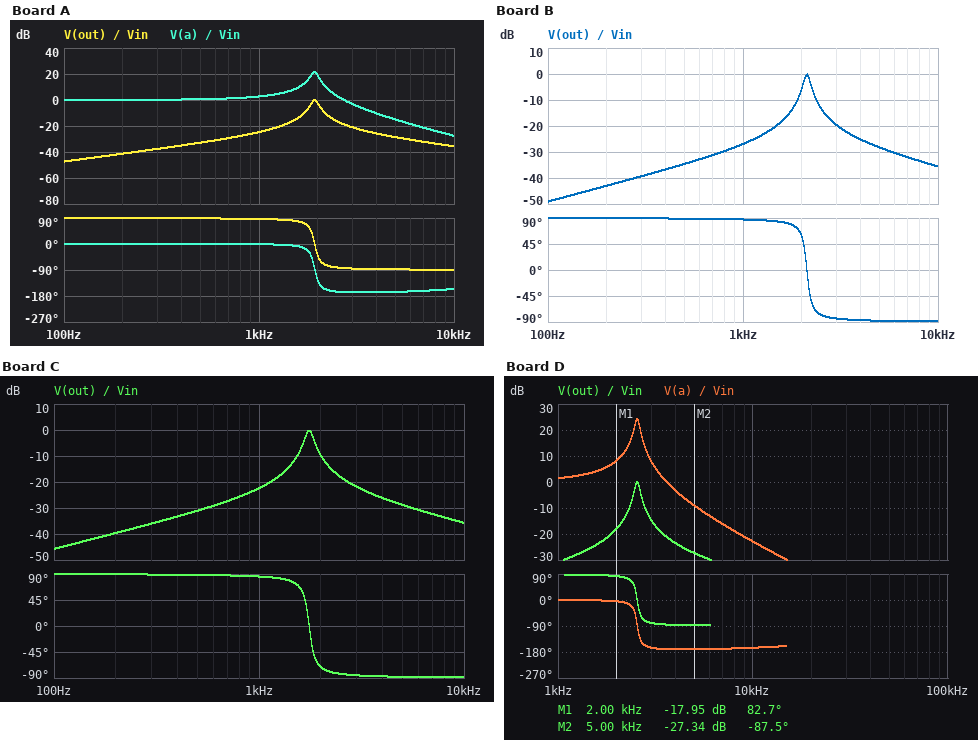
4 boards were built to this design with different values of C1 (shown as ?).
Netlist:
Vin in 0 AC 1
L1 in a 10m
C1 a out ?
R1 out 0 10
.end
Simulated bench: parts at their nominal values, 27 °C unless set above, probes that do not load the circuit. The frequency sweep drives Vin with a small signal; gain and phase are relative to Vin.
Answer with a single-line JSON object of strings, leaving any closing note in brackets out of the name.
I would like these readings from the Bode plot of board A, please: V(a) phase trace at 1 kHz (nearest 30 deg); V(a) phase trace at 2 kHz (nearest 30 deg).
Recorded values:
{"V(a) phase trace at 1 kHz": "0 deg", "V(a) phase trace at 2 kHz": "-120 deg"}
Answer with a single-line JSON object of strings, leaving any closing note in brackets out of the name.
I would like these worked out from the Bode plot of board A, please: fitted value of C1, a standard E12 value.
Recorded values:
{"fitted value of C1, a standard E12 value": "680 nF"}
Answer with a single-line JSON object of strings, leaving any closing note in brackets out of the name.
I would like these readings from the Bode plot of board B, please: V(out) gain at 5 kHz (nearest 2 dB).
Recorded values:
{"V(out) gain at 5 kHz": "-28 dB"}
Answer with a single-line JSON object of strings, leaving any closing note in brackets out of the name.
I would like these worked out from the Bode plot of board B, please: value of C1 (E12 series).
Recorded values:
{"value of C1": "560 nF"}
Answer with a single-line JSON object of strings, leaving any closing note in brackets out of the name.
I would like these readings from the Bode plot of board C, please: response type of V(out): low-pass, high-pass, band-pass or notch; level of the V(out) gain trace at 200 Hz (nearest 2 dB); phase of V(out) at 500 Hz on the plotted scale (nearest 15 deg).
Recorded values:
{"response type of V(out): low-pass, high-pass, band-pass or notch": "band-pass", "level of the V(out) gain trace at 200 Hz": "-40 dB", "phase of V(out) at 500 Hz on the plotted scale": "90 deg"}
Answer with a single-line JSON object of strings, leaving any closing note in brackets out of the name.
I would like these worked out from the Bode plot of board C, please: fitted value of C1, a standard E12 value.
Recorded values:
{"fitted value of C1, a standard E12 value": "820 nF"}
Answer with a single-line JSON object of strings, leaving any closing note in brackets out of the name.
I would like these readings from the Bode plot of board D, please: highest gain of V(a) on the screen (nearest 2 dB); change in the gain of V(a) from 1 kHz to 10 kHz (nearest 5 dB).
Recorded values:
{"highest gain of V(a) on the screen": "24 dB", "change in the gain of V(a) from 1 kHz to 10 kHz": "-25 dB"}
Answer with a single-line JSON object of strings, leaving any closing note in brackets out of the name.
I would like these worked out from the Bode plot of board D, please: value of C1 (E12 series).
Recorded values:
{"value of C1": "390 nF"}
